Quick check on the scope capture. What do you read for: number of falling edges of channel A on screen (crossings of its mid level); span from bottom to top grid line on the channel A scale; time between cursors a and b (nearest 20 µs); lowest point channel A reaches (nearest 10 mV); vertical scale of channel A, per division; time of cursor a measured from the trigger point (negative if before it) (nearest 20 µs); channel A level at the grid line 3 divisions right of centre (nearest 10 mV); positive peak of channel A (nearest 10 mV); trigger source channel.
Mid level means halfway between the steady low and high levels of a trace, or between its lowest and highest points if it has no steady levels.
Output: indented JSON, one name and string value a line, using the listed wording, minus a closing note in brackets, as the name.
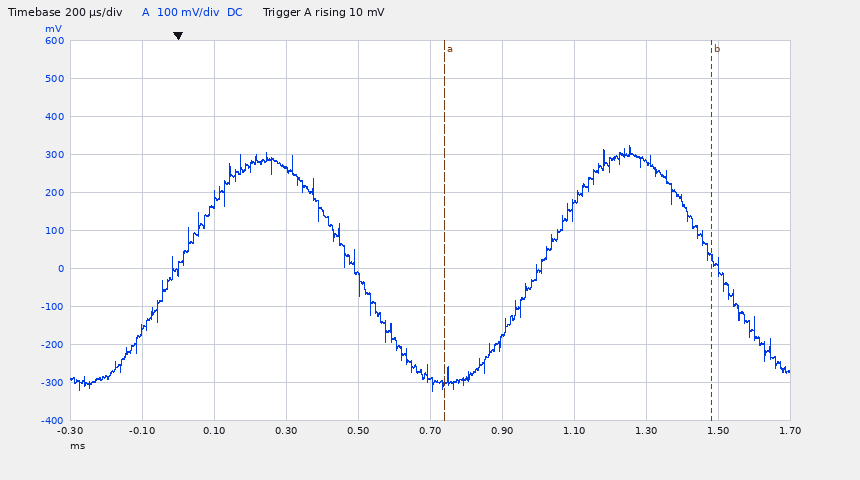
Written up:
{
  "number of falling edges of channel A on screen": "2",
  "span from bottom to top grid line on the channel A scale": "1 V",
  "time between cursors a and b": "740 µs",
  "lowest point channel A reaches": "-320 mV",
  "vertical scale of channel A, per division": "100 mV",
  "time of cursor a measured from the trigger point (negative if before it)": "+740 µs",
  "channel A level at the grid line 3 divisions right of centre": "280 mV",
  "positive peak of channel A": "320 mV",
  "trigger source channel": "channel A"
}
